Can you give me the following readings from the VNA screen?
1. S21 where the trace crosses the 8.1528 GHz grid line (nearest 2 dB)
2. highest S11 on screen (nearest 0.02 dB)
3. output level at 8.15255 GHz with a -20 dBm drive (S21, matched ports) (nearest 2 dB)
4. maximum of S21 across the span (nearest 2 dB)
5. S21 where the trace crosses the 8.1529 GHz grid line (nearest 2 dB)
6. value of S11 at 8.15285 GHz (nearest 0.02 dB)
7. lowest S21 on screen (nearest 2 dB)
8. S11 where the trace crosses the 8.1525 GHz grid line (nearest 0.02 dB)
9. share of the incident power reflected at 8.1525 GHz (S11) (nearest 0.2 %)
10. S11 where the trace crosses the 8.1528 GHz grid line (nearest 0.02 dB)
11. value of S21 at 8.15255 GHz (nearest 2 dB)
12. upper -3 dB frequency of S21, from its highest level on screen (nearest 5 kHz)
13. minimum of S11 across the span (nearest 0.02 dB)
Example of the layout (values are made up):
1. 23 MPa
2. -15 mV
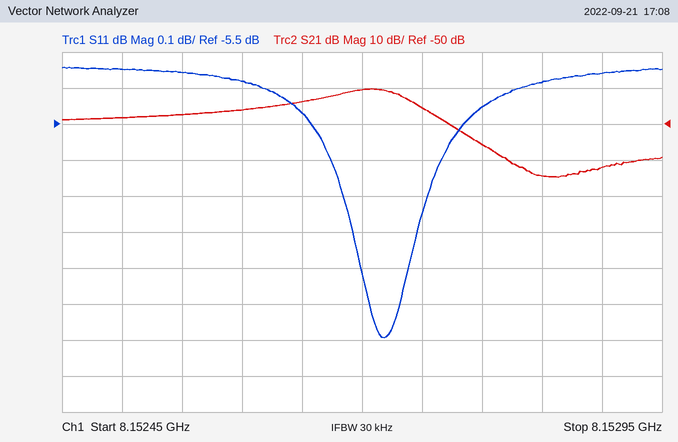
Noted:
1. -56 dB
2. -5.34 dB
3. -68 dBm
4. -40 dB
5. -62 dB
6. -5.38 dB
7. -64 dB
8. -5.34 dB
9. 29.2 %
10. -5.46 dB
11. -48 dB
12. 8.152740 GHz
13. -6.10 dB
